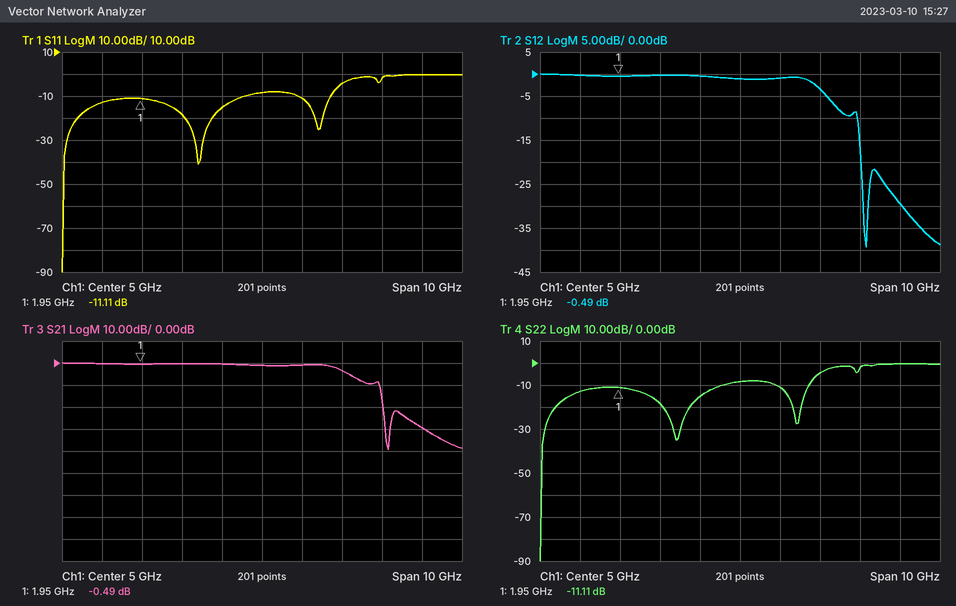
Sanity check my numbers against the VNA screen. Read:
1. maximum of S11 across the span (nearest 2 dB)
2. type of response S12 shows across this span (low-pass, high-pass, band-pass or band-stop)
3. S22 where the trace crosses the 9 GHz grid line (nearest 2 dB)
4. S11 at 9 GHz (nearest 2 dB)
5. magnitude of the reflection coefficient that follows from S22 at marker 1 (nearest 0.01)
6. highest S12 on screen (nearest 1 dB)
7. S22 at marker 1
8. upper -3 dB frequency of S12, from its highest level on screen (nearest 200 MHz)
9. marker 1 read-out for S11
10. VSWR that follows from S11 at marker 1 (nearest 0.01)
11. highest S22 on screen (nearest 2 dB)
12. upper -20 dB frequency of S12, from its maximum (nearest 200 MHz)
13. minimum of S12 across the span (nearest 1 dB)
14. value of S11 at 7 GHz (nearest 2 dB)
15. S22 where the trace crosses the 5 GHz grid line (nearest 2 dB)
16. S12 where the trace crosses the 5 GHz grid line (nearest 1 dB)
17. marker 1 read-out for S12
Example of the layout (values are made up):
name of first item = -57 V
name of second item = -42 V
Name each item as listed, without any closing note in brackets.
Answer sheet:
maximum of S11 across the span = 0 dB
type of response S12 shows across this span = low-pass
S22 where the trace crosses the 9 GHz grid line = 0 dB
S11 at 9 GHz = 0 dB
magnitude of the reflection coefficient that follows from S22 at marker 1 = 0.28
highest S12 on screen = 0 dB
S22 at marker 1 = -11.11 dB
upper -3 dB frequency of S12, from its highest level on screen = 7.0 GHz
marker 1 read-out for S11 = -11.11 dB
VSWR that follows from S11 at marker 1 = 1.77
highest S22 on screen = 0 dB
upper -20 dB frequency of S12, from its maximum = 8.0 GHz
minimum of S12 across the span = -39 dB
value of S11 at 7 GHz = -4 dB
S22 where the trace crosses the 5 GHz grid line = -8 dB
S12 where the trace crosses the 5 GHz grid line = -1 dB
marker 1 read-out for S12 = -0.49 dB
